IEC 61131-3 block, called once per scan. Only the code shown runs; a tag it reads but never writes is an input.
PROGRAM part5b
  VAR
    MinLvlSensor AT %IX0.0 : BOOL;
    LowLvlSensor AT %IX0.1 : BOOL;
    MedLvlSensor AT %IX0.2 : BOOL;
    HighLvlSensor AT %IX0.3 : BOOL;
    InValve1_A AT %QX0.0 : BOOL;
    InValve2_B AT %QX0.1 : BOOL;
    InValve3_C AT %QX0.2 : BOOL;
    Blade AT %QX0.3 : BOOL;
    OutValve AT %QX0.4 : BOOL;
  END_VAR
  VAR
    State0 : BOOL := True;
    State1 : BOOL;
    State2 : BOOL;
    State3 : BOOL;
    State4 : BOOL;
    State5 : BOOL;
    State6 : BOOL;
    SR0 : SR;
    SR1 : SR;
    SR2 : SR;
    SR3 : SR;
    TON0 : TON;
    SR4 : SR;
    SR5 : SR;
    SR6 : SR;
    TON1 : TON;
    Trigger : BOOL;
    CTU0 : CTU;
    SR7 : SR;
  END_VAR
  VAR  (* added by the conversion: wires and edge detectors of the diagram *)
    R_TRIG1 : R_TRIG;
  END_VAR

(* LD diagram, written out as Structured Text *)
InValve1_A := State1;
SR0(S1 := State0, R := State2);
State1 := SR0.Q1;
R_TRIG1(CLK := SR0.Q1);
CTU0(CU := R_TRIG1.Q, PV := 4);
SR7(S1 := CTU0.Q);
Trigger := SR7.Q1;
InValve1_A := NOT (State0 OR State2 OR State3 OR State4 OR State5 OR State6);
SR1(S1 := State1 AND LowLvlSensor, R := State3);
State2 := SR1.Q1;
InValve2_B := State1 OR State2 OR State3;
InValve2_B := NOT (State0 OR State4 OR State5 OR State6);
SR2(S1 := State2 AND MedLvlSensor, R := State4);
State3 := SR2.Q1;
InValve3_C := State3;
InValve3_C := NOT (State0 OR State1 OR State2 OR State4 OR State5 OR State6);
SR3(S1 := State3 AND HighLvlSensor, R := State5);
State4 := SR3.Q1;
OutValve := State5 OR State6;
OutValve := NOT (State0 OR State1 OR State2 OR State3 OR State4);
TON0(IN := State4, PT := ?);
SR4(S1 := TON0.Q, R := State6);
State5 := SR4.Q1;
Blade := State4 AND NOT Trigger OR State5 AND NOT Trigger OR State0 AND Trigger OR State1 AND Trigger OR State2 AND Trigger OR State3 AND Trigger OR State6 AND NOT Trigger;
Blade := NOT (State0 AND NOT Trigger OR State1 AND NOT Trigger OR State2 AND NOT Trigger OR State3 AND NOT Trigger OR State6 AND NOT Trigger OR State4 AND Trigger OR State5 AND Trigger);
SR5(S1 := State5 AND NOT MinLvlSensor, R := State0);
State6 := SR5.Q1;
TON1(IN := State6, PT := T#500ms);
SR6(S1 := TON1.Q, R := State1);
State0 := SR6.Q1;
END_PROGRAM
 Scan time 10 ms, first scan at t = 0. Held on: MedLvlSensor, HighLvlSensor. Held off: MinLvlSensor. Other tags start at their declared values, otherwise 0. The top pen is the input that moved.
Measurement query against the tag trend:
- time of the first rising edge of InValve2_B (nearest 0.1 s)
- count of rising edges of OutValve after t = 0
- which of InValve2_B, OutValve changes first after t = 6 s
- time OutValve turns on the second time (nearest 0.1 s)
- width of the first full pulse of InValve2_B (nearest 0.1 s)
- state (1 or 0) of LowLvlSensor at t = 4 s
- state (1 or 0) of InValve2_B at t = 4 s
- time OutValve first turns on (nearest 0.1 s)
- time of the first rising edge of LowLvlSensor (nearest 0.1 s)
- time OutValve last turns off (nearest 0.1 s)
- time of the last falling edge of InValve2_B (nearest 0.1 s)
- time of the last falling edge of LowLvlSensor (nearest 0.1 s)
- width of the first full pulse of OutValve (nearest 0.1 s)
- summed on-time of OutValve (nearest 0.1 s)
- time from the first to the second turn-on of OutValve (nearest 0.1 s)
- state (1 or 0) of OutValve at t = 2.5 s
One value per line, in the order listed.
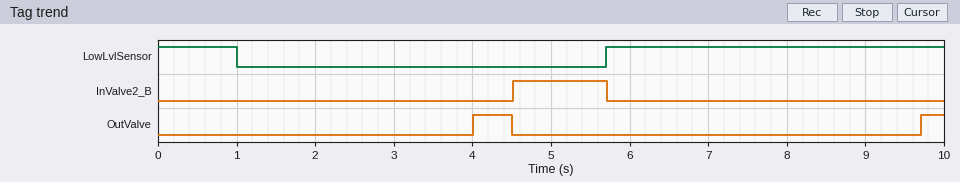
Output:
4.5 s
2
OutValve
9.7 s
1.2 s
0
0
4.0 s
5.7 s
4.5 s
5.7 s
1.0 s
0.5 s
0.8 s
5.7 s
0
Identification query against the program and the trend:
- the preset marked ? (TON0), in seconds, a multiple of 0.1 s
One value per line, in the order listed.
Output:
4.0 s
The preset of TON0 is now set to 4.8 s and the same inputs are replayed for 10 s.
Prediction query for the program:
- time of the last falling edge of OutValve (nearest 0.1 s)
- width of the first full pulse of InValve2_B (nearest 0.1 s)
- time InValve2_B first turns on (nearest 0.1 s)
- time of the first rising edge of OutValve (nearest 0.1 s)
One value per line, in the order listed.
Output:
5.3 s
0.4 s
5.3 s
4.8 s
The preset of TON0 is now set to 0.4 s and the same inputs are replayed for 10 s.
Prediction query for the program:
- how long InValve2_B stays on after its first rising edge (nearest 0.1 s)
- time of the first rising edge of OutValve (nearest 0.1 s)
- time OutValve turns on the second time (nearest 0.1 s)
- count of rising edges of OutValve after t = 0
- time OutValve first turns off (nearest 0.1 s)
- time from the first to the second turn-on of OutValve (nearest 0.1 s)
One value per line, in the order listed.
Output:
3.9 s
0.4 s
1.3 s
7
0.9 s
0.9 s
